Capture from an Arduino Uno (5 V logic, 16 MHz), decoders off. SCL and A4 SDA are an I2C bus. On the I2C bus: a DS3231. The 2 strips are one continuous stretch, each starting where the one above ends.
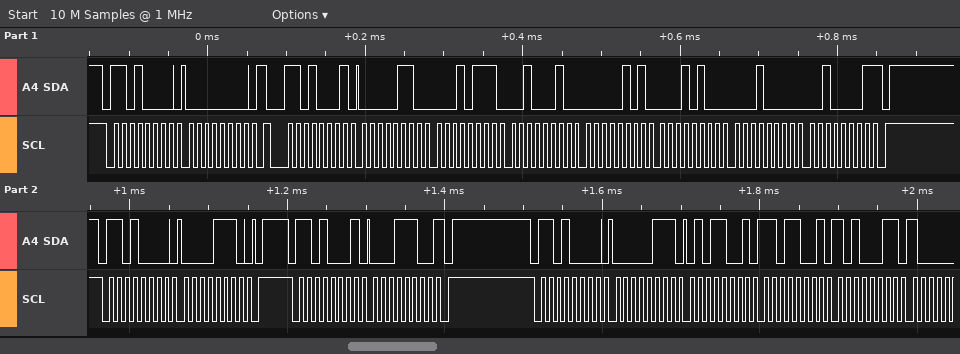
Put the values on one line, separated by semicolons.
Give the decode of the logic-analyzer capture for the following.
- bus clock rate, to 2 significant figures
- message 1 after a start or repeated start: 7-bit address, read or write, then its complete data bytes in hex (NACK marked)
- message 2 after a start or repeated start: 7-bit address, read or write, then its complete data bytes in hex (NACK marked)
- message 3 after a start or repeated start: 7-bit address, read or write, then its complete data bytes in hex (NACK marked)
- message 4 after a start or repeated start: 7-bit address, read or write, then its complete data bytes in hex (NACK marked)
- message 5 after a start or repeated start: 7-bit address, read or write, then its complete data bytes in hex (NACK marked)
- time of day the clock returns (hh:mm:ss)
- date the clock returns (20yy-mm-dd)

100 kHz; 0x68 write: 00; 0x68 read: 06 17 22 05 14 10 21 NACK; 0x68 write: 0E; 0x68 read: 1C NACK; 0x68 write: 07 59 D9 A3; 22:17:06; 2021-10-14
